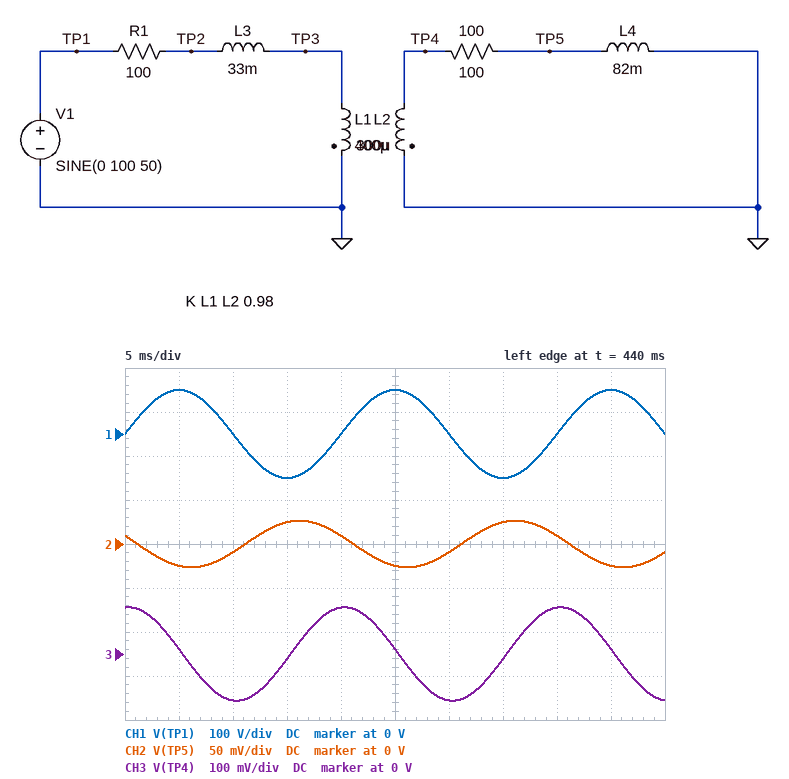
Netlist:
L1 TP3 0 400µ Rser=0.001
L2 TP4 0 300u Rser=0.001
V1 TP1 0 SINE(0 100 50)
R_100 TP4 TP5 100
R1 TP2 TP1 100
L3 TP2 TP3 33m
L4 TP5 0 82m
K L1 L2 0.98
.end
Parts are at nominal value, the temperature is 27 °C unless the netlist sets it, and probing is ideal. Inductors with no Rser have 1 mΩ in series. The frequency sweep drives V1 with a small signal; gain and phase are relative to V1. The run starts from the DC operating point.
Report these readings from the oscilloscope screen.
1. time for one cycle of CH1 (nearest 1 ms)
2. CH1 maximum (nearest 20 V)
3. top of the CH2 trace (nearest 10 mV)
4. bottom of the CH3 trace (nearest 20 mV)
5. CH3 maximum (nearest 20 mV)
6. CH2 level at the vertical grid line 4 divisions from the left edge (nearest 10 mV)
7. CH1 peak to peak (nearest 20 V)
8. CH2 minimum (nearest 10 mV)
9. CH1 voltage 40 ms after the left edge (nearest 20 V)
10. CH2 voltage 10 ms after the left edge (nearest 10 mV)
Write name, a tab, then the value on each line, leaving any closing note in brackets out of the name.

time for one cycle of CH1	20 ms
CH1 maximum	100 V
top of the CH2 trace	30 mV
bottom of the CH3 trace	-100 mV
CH3 maximum	100 mV
CH2 level at the vertical grid line 4 divisions from the left edge	10 mV
CH1 peak to peak	200 V
CH2 minimum	-30 mV
CH1 voltage 40 ms after the left edge	0 V
CH2 voltage 10 ms after the left edge	-10 mV
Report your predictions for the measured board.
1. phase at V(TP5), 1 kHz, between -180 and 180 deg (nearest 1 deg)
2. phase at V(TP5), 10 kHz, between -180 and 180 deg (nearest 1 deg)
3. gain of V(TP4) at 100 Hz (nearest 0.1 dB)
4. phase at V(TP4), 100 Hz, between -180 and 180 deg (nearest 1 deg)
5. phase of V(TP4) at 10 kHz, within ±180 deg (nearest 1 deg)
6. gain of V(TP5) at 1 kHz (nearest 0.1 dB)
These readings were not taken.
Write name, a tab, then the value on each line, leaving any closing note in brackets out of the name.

phase at V(TP5), 1 kHz, between -180 and 180 deg	36 deg
phase at V(TP5), 10 kHz, between -180 and 180 deg	4 deg
gain of V(TP4) at 100 Hz	-53.6 dB
phase at V(TP4), 100 Hz, between -180 and 180 deg	78 deg
phase of V(TP4) at 10 kHz, within ±180 deg	3 deg
gain of V(TP5) at 1 kHz	-40.9 dB
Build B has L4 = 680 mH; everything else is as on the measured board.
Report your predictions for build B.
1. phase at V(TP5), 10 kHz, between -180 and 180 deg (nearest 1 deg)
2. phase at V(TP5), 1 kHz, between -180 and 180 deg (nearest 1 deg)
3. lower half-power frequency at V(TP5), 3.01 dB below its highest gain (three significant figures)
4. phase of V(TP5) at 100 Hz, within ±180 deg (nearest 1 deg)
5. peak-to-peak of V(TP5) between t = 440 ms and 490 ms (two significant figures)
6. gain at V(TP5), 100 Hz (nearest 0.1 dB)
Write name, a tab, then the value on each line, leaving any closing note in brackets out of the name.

phase at V(TP5), 10 kHz, between -180 and 180 deg	3 deg
phase at V(TP5), 1 kHz, between -180 and 180 deg	27 deg
lower half-power frequency at V(TP5), 3.01 dB below its highest gain	478 Hz
phase of V(TP5) at 100 Hz, within ±180 deg	91 deg
peak-to-peak of V(TP5) between t = 440 ms and 490 ms	190 mV
gain at V(TP5), 100 Hz	-53.8 dB
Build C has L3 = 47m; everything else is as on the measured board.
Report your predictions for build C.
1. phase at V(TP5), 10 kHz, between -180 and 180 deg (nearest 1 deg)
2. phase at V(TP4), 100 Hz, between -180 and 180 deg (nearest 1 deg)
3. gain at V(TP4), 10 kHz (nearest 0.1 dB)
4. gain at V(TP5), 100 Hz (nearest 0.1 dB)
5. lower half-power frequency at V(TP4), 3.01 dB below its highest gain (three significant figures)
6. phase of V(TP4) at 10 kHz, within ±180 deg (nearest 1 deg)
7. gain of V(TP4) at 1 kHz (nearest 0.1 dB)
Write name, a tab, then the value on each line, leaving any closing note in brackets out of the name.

phase at V(TP5), 10 kHz, between -180 and 180 deg	3 deg
phase at V(TP4), 100 Hz, between -180 and 180 deg	73 deg
gain at V(TP4), 10 kHz	-42.9 dB
gain at V(TP5), 100 Hz	-60.6 dB
lower half-power frequency at V(TP4), 3.01 dB below its highest gain	335 Hz
phase of V(TP4) at 10 kHz, within ±180 deg	2 deg
gain of V(TP4) at 1 kHz	-43.4 dB
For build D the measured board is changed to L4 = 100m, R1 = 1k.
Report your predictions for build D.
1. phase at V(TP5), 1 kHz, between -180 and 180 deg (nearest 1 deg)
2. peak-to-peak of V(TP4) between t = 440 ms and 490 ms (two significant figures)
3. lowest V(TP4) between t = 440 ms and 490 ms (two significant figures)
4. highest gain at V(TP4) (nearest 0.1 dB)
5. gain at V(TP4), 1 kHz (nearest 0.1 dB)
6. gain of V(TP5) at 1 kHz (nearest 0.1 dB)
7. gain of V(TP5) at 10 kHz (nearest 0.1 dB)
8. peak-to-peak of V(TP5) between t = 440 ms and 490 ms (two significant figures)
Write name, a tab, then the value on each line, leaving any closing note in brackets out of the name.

phase at V(TP5), 1 kHz, between -180 and 180 deg	87 deg
peak-to-peak of V(TP4) between t = 440 ms and 490 ms	21 mV
lowest V(TP4) between t = 440 ms and 490 ms	-11 mV
highest gain at V(TP4)	-39.9 dB
gain at V(TP4), 1 kHz	-53.6 dB
gain of V(TP5) at 1 kHz	-53.7 dB
gain of V(TP5) at 10 kHz	-40.8 dB
peak-to-peak of V(TP5) between t = 440 ms and 490 ms	6.4 mV
